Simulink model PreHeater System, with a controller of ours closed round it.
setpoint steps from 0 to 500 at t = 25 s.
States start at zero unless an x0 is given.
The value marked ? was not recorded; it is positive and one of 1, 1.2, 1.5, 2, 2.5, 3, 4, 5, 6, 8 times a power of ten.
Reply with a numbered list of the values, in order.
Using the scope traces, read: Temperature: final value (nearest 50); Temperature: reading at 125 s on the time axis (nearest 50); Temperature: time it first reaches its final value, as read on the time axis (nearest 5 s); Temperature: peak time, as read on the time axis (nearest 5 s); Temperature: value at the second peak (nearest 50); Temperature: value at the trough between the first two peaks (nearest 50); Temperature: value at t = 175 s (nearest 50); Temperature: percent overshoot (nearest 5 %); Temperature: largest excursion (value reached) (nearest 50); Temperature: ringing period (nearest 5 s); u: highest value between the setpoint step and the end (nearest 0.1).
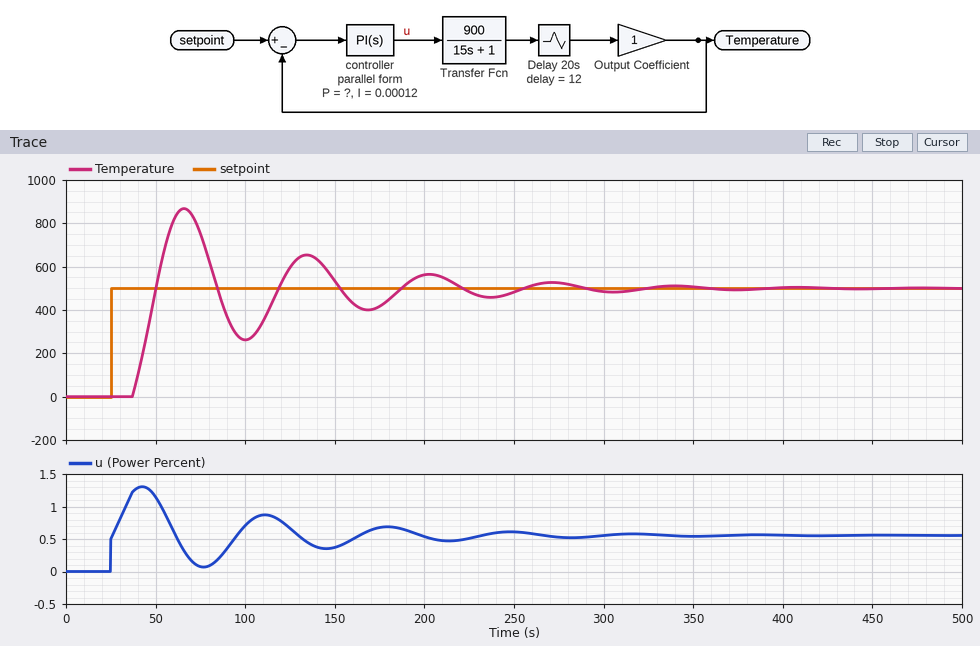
1. 500
2. 600
3. 50 s
4. 65 s
5. 650
6. 250
7. 400
8. 75 %
9. 850
10. 70 s
11. 1.3
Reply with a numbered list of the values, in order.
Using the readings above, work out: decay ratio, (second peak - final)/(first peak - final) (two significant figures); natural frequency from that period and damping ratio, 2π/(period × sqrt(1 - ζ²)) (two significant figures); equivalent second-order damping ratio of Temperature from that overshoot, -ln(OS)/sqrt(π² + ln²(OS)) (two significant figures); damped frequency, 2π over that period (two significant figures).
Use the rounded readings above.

1. 0.43
2. 0.090 rad/s
3. 0.091
4. 0.090 rad/s
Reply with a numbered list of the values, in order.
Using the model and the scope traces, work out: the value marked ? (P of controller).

1. 0.001
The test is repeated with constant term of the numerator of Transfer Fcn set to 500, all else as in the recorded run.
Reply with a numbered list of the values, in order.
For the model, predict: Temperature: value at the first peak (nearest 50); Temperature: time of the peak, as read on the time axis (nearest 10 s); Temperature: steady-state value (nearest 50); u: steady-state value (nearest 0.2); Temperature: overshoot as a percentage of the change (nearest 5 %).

1. 650
2. 80 s
3. 500
4. 1.0
5. 30 %
